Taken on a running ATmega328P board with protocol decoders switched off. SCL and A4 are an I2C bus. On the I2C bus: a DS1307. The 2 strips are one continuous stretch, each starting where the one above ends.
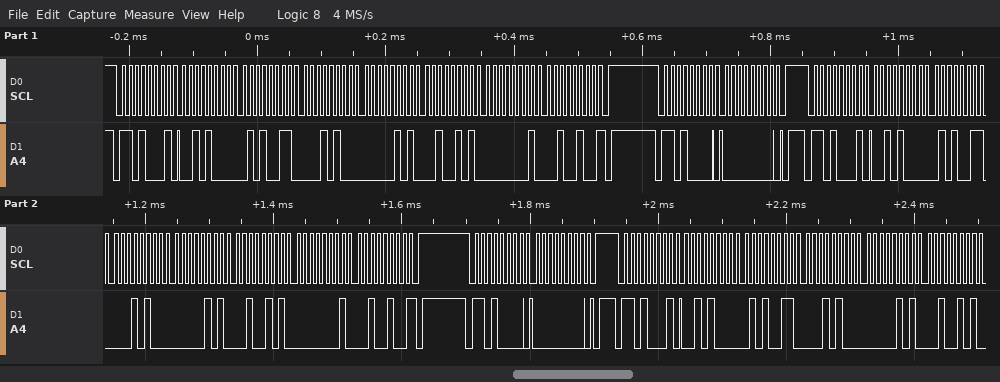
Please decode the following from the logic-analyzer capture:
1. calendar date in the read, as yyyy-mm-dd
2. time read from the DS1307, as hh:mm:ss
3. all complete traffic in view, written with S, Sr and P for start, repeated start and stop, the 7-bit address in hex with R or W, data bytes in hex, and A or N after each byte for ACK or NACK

2024-01-25
14:53:28
S 68R A 28 A 53 A 14 A 05 A 25 A 01 A 24 N P S 68W A 00 A P S 68R A 28 A 53 A 14 A 05 A 25 A 01 A 24 N P S 68W A 00 A P S 68R A 28 A 53 A 14 A 05 A 25 A
